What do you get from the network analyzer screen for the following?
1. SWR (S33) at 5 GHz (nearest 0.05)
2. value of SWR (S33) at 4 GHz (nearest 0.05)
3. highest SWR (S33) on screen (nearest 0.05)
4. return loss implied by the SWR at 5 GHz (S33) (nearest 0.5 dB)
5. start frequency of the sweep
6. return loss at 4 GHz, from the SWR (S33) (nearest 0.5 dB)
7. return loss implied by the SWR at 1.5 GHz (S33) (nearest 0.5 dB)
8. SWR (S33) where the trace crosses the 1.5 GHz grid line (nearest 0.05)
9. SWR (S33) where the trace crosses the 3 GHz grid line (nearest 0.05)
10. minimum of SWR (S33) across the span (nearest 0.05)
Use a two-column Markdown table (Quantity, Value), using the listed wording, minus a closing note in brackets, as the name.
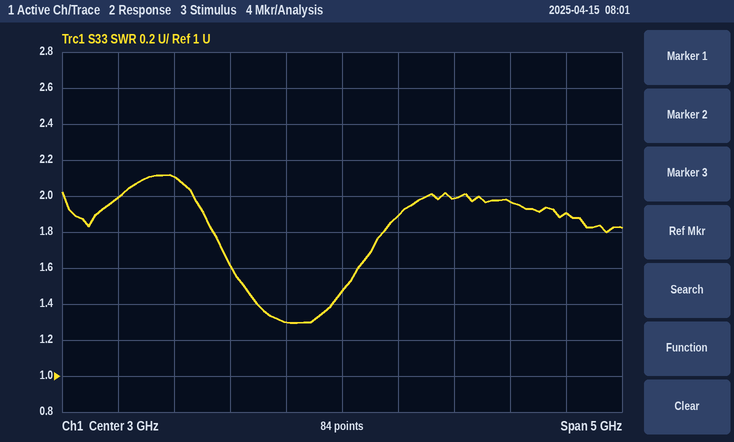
| Quantity | Value |
|---|---|
| SWR (S33) at 5 GHz | 1.90 |
| value of SWR (S33) at 4 GHz | 2.00 |
| highest SWR (S33) on screen | 2.10 |
| return loss implied by the SWR at 5 GHz (S33) | 10.0 dB |
| start frequency of the sweep | 500 MHz |
| return loss at 4 GHz, from the SWR (S33) | 9.5 dB |
| return loss implied by the SWR at 1.5 GHz (S33) | 9.0 dB |
| SWR (S33) where the trace crosses the 1.5 GHz grid line | 2.10 |
| SWR (S33) where the trace crosses the 3 GHz grid line | 1.45 |
| minimum of SWR (S33) across the span | 1.30 |
